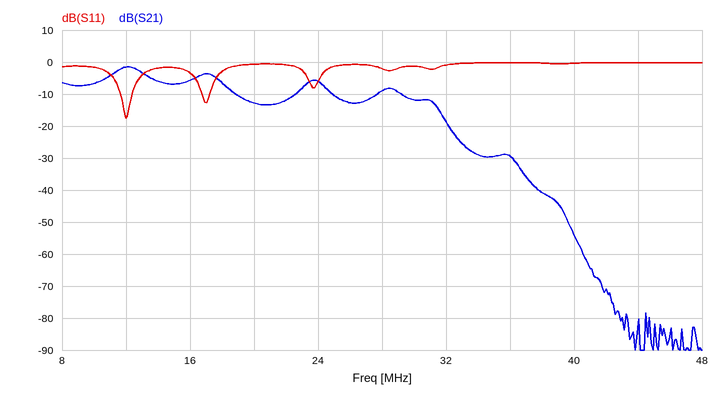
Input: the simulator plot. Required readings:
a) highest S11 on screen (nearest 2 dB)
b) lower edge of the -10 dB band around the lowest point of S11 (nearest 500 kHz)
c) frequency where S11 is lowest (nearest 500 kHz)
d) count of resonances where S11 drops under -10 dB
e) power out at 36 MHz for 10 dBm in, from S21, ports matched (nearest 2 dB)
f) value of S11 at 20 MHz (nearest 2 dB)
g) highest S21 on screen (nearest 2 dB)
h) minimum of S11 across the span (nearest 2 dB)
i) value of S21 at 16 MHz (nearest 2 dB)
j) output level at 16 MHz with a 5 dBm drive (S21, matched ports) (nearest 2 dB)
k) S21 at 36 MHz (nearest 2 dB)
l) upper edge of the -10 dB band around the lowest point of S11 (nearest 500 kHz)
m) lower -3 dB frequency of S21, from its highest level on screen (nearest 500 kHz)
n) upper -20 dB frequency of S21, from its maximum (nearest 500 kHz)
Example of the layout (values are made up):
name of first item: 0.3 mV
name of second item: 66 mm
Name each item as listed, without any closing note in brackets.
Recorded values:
highest S11 on screen: 0 dB
lower edge of the -10 dB band around the lowest point of S11: 11.5 MHz
frequency where S11 is lowest: 12.0 MHz
count of resonances where S11 drops under -10 dB: 2
power out at 36 MHz for 10 dBm in, from S21, ports matched: -20 dBm
value of S11 at 20 MHz: 0 dB
highest S21 on screen: -2 dB
minimum of S11 across the span: -18 dB
value of S21 at 16 MHz: -6 dB
output level at 16 MHz with a 5 dBm drive (S21, matched ports): 0 dBm
S21 at 36 MHz: -30 dB
upper edge of the -10 dB band around the lowest point of S11: 12.5 MHz
lower -3 dB frequency of S21, from its highest level on screen: 11.0 MHz
upper -20 dB frequency of S21, from its maximum: 32.5 MHz
